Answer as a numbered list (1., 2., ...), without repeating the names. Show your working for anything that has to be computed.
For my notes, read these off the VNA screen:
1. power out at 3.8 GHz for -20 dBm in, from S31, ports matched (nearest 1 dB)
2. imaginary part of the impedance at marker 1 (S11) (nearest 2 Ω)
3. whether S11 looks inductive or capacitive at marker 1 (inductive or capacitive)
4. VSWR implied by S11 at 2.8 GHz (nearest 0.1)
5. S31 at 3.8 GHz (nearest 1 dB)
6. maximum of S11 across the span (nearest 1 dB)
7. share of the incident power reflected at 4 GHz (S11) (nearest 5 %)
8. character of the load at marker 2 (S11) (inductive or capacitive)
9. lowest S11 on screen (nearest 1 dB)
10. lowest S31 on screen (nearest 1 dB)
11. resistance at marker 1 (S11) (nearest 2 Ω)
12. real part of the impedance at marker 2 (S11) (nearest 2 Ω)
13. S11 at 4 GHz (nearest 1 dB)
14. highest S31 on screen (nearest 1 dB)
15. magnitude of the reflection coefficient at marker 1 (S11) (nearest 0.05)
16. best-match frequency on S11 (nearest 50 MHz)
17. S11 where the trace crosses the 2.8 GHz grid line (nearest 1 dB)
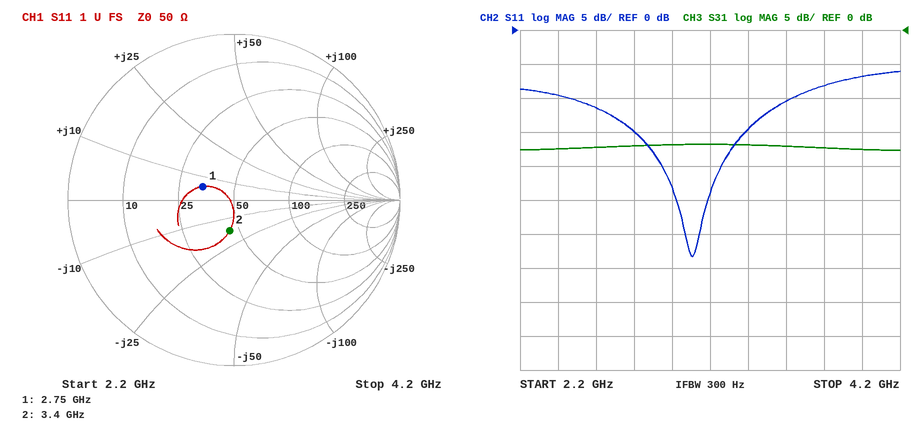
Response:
1. -20 dBm + (-17 dB) = -37 dBm
2. +6 Ω
3. inductive
4. |Γ| = 10^(-15/20) = 0.1778; VSWR = (1 + 0.1778)/(1 − 0.1778) ≈ 1.4
5. -17 dB
6. -6 dB
7. 10^(-7/10) ≈ 20 %
8. capacitive
9. -33 dB
10. -18 dB
11. 34 Ω
12. 44 Ω
13. -7 dB
14. -17 dB
15. 0.20
16. 3.10 GHz
17. -15 dB
